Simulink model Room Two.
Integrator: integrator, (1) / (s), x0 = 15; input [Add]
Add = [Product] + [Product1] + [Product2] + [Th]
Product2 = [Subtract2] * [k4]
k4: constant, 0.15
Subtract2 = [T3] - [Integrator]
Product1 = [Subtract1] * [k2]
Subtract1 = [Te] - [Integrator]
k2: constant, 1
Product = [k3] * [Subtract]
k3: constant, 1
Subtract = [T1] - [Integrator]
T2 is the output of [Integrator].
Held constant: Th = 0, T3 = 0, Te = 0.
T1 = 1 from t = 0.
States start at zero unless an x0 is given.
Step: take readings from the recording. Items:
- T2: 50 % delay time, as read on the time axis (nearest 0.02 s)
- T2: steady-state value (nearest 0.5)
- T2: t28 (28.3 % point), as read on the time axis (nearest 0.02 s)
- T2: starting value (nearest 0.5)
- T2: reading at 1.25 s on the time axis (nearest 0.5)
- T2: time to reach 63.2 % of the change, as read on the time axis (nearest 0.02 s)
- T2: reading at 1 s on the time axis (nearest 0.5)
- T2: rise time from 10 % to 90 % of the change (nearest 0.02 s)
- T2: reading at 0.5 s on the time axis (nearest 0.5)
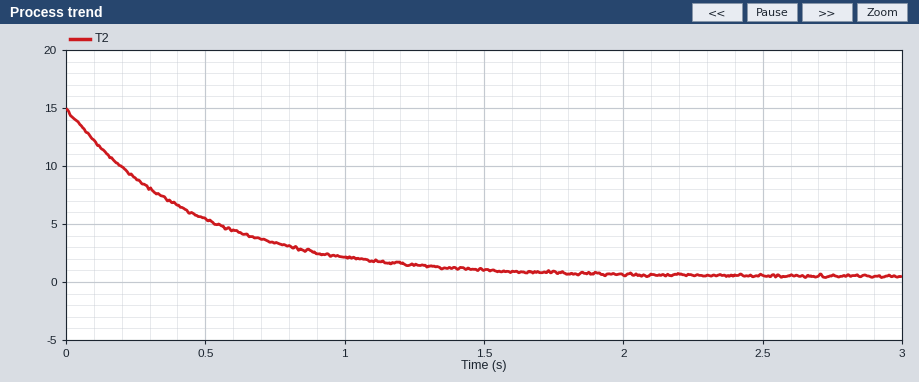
0.32 s
0.5
0.16 s
15.0
1.5
0.46 s
2.0
1.02 s
5.5
